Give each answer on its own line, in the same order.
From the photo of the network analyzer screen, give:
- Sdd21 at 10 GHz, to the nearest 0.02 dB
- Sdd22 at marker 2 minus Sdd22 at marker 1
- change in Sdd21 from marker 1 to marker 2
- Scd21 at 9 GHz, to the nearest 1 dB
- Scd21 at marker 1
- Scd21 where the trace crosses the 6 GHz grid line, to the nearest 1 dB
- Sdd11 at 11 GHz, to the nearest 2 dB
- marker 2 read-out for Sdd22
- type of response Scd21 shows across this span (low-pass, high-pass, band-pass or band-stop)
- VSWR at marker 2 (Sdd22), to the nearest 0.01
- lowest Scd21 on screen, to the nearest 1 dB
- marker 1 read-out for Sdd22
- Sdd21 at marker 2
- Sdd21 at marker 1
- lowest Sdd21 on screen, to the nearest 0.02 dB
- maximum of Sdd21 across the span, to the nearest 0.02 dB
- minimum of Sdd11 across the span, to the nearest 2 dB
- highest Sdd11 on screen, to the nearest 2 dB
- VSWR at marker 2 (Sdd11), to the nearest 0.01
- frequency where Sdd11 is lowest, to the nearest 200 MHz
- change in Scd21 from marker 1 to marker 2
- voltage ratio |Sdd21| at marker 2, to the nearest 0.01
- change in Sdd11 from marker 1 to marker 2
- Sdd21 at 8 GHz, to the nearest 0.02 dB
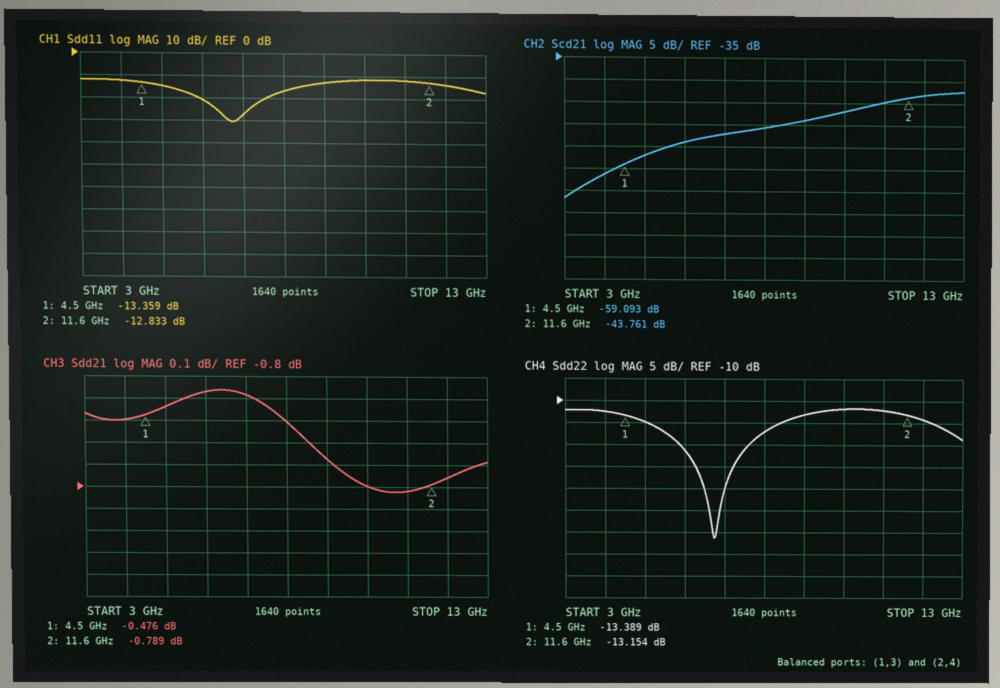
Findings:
-0.80 dB
0.235 dB
-0.313 dB
-49 dB
-59.093 dB
-54 dB
-12 dB
-13.154 dB
high-pass
1.56
-67 dB
-13.389 dB
-0.789 dB
-0.476 dB
-0.82 dB
-0.36 dB
-30 dB
-12 dB
1.59
6.8 GHz
15.332 dB
0.91
0.526 dB
-0.50 dB
